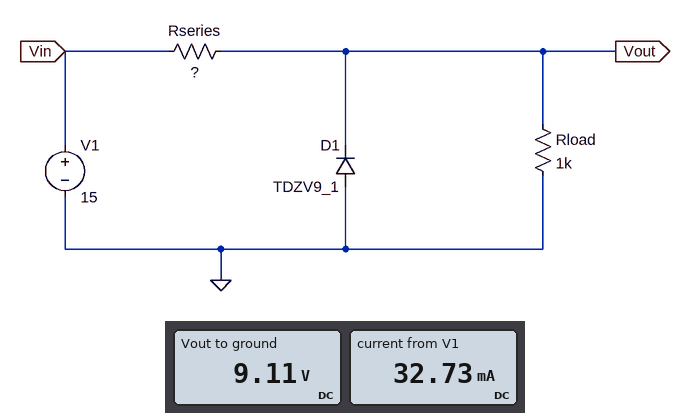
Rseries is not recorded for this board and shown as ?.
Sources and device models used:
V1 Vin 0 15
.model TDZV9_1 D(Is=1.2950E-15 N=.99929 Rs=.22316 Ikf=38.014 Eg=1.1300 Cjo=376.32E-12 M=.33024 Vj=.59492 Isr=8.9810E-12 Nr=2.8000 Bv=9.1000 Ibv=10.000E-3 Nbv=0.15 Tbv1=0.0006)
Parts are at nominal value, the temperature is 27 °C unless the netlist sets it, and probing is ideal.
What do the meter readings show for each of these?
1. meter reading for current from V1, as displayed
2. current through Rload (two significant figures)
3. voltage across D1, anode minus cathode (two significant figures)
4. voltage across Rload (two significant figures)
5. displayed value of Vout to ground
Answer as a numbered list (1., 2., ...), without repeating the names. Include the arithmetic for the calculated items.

1. 32.73 mA
2. (9.11 V) / 1 kΩ = 9.1 mA
3. 0 V - 9.11 V = -9.1 V
4. 9.11 V = 9.1 V
5. 9.11 V
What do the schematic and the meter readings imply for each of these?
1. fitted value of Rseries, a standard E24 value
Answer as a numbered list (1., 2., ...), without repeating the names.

1. 180 Ω
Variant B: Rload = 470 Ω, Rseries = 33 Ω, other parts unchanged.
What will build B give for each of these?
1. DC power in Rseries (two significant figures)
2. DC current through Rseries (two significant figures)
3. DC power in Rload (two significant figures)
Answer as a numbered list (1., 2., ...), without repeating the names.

1. 1.0 W
2. 180 mA
3. 180 mW
